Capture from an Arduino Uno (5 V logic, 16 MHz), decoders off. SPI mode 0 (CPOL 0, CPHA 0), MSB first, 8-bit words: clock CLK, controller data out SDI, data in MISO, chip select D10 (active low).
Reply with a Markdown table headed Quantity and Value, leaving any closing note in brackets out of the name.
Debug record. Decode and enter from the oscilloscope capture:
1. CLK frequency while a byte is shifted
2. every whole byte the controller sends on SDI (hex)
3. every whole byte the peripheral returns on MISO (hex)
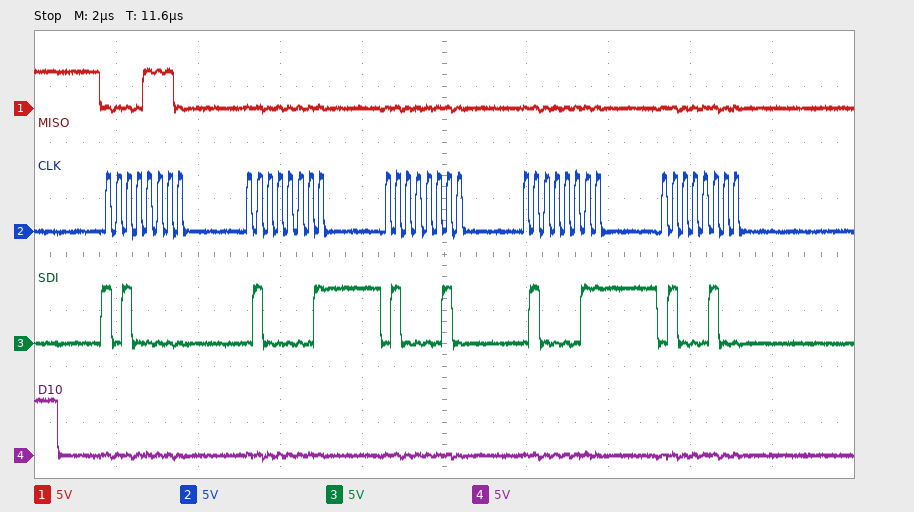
| Quantity | Value |
|---|---|
| CLK frequency while a byte is shifted | 4 MHz |
| every whole byte the controller sends on SDI | A0 41 42 43 44 |
| every whole byte the peripheral returns on MISO | 0E 00 00 00 00 |
